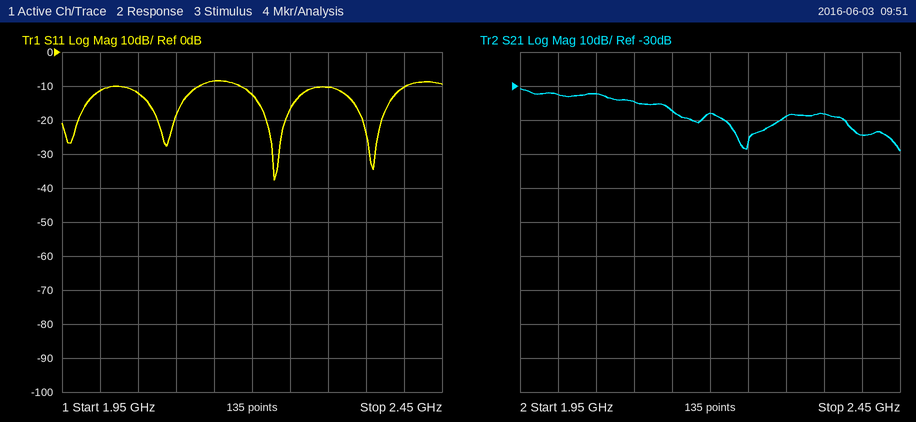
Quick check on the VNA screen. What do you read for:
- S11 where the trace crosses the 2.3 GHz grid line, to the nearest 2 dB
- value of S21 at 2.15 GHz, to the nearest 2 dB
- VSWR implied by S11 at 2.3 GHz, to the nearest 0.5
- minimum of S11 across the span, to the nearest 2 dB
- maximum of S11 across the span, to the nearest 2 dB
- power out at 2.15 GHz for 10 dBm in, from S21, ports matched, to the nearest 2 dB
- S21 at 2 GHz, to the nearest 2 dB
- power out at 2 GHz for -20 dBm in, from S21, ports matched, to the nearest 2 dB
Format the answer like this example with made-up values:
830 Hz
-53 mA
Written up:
-10 dB
-38 dB
2.0
-38 dB
-8 dB
-28 dBm
-32 dB
-52 dBm
